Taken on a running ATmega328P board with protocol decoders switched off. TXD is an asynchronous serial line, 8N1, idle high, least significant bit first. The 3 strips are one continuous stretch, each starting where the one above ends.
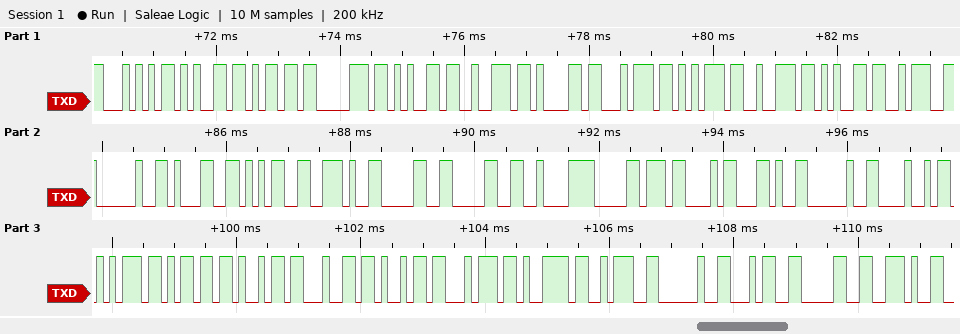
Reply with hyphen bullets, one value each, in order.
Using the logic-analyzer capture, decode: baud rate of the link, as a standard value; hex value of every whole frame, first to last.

- 9600 baud
- 54 65 6D 70 65 72 61 74 75 72 65 3A 20 31 35 2E 30 30 C2 B0 43 2C 20 48 75 6D 69 64 69 74 79 3A 20 34 30 2E
